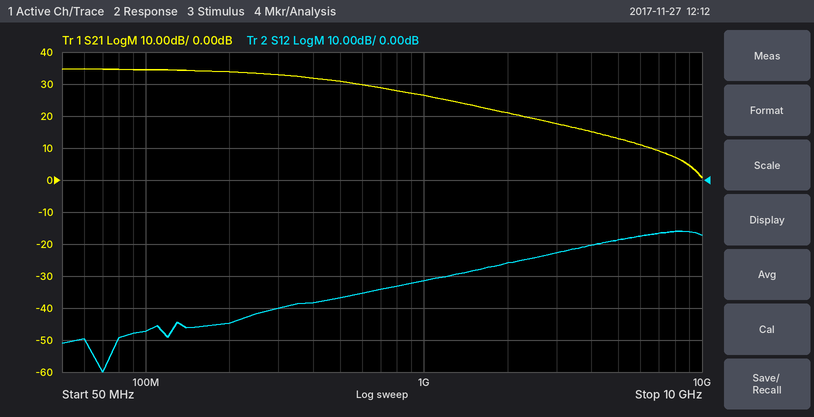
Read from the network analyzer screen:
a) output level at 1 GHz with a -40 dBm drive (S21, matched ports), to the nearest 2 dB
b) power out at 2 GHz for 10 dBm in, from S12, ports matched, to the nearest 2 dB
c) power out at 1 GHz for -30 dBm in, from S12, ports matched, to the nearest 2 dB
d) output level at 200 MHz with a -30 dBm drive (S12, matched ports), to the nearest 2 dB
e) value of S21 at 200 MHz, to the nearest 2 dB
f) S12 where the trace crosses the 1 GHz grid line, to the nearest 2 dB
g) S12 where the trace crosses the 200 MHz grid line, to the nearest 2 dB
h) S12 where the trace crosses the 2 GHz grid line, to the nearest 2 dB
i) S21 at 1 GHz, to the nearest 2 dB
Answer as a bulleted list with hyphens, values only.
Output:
- -14 dBm
- -16 dBm
- -62 dBm
- -74 dBm
- 34 dB
- -32 dB
- -44 dB
- -26 dB
- 26 dB
